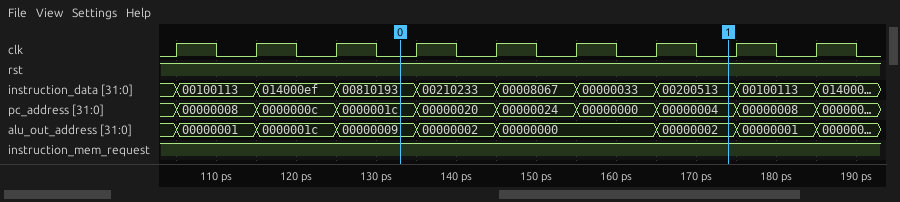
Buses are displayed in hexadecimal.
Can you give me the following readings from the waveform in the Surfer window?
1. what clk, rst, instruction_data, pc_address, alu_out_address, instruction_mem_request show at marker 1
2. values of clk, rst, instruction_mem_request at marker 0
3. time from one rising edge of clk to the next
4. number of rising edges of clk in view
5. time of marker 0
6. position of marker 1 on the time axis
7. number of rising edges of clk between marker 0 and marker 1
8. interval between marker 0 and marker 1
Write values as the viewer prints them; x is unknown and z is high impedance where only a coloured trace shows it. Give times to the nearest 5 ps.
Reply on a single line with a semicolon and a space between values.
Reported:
clk=0, rst=1, instruction_data=00200513, pc_address=00000004, alu_out_address=00000002, instruction_mem_request=1; clk=0, rst=1, instruction_mem_request=1; 10 ps; 9; 135 ps; 175 ps; 4; 40 ps
